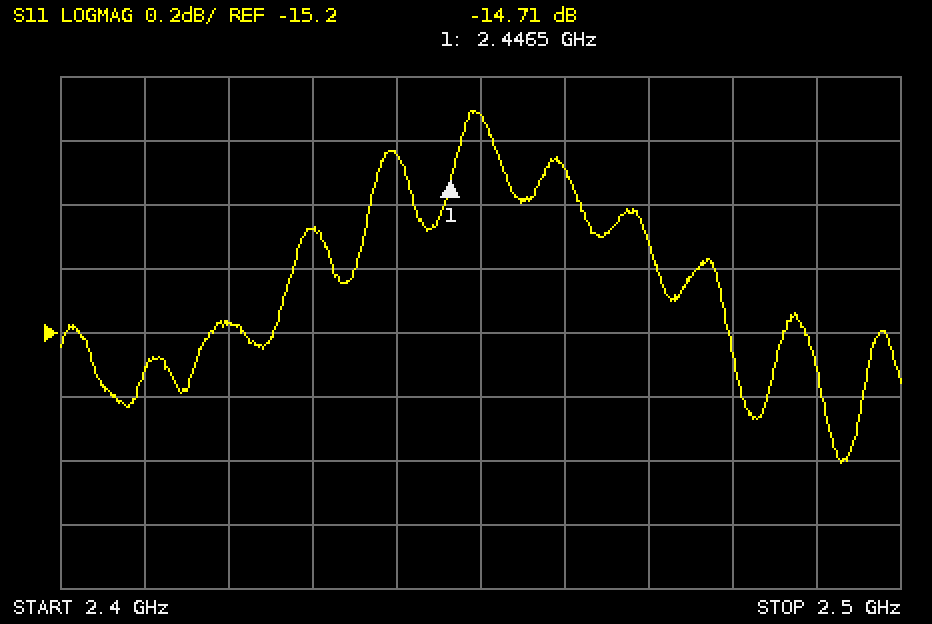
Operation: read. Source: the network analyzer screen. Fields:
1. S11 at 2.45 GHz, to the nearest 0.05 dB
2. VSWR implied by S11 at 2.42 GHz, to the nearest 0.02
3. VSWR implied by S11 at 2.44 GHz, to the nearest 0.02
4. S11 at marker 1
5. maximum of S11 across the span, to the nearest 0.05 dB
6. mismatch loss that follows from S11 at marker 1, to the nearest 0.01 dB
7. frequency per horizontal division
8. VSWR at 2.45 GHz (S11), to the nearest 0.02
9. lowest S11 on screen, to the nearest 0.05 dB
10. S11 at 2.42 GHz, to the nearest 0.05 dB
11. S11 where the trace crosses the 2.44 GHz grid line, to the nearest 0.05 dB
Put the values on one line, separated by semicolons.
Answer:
-14.50 dB; 1.42; 1.46; -14.71 dB; -14.50 dB; 0.15 dB; 10 MHz; 1.46; -15.60 dB; -15.15 dB; -14.65 dB
